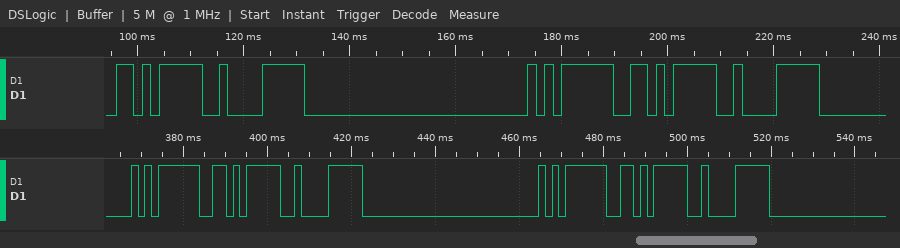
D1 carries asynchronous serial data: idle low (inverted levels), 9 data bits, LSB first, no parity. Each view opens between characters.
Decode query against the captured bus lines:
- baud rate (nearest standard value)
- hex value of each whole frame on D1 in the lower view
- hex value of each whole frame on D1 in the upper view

600 baud
05, 0A, 0F, 05, 0A, 0F
0A, 0F, 05, 0A, 0F
